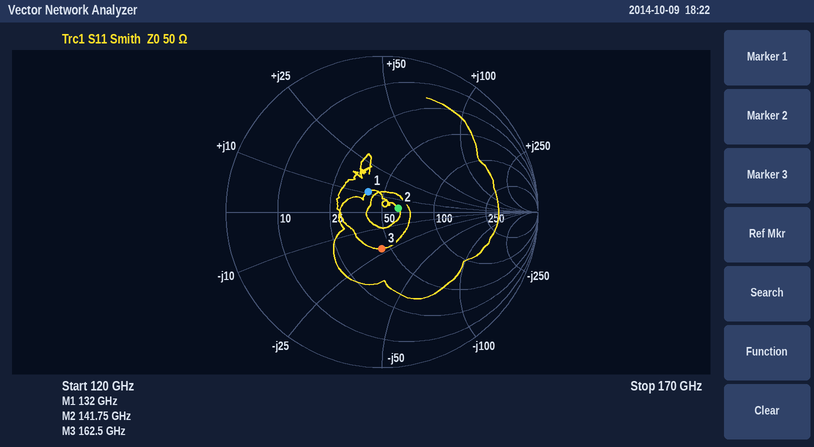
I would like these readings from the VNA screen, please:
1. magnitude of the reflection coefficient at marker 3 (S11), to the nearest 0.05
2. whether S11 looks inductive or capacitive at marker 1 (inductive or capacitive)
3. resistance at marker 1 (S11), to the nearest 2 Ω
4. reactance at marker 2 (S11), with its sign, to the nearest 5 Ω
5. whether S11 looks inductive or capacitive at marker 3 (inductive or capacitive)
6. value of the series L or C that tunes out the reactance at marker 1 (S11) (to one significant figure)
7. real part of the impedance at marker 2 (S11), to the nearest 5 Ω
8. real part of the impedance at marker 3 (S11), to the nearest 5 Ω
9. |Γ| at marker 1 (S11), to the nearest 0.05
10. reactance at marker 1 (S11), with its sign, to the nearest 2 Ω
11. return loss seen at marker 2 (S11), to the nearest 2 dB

0.25
inductive
40 Ω
+5 Ω
capacitive
100 fF
60 Ω
45 Ω
0.15
+10 Ω
20 dB
